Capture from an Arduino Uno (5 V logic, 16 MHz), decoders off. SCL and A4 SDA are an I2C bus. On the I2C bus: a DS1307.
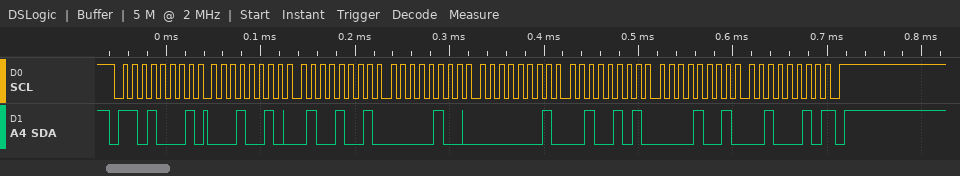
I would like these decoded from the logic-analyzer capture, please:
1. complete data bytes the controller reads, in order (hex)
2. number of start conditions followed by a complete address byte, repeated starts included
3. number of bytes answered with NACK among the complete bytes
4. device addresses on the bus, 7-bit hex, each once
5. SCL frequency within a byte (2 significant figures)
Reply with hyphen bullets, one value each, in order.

- 12 49 04 01 25 09 22
- 1
- 1
- 0x68
- 100 kHz
